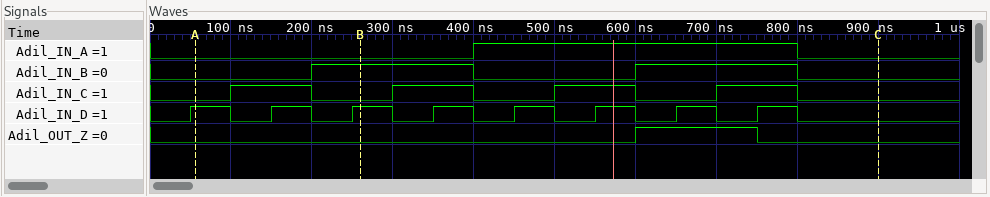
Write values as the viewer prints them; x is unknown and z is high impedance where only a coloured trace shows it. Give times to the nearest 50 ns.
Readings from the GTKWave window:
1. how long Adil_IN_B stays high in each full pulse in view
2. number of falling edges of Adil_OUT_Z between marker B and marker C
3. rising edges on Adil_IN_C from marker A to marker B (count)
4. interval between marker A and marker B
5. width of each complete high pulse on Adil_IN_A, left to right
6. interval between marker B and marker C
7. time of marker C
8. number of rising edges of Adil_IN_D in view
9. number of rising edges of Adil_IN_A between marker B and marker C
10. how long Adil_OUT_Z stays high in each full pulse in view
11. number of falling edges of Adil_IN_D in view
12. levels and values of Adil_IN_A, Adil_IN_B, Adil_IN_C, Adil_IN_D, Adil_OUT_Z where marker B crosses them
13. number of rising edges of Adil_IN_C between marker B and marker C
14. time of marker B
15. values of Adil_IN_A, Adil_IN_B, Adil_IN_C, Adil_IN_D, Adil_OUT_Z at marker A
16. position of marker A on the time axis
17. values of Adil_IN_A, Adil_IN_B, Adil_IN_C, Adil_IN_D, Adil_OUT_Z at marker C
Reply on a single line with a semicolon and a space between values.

200 ns, 200 ns; 1; 1; 200 ns; 400 ns; 650 ns; 900 ns; 8; 1; 150 ns; 8; Adil_IN_A=0, Adil_IN_B=1, Adil_IN_C=0, Adil_IN_D=1, Adil_OUT_Z=0; 3; 250 ns; Adil_IN_A=0, Adil_IN_B=0, Adil_IN_C=0, Adil_IN_D=1, Adil_OUT_Z=0; 50 ns; Adil_IN_A=0, Adil_IN_B=0, Adil_IN_C=0, Adil_IN_D=0, Adil_OUT_Z=0
